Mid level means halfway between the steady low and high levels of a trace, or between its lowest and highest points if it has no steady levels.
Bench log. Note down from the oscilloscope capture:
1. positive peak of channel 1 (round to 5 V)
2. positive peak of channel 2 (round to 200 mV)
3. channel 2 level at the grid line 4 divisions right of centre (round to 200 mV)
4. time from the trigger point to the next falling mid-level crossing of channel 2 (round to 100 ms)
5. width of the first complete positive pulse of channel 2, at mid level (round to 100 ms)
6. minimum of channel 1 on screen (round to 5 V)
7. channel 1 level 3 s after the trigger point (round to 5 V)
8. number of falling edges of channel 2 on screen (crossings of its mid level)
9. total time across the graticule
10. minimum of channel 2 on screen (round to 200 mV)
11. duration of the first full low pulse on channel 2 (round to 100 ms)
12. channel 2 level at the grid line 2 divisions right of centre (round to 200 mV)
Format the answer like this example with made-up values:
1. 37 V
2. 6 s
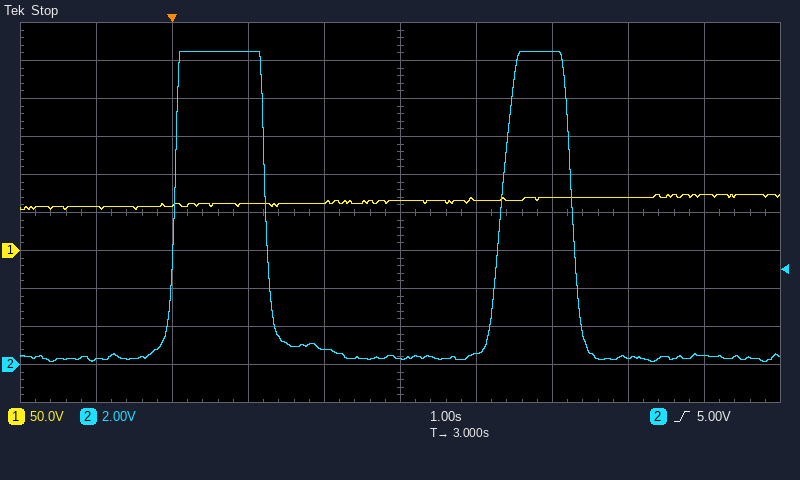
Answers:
1. 75 V
2. 16.4 V
3. 400 mV
4. 1.2 s
5. 1.2 s
6. 55 V
7. 65 V
8. 2
9. 10 s
10. 200 mV
11. 3.1 s
12. 16.4 V
